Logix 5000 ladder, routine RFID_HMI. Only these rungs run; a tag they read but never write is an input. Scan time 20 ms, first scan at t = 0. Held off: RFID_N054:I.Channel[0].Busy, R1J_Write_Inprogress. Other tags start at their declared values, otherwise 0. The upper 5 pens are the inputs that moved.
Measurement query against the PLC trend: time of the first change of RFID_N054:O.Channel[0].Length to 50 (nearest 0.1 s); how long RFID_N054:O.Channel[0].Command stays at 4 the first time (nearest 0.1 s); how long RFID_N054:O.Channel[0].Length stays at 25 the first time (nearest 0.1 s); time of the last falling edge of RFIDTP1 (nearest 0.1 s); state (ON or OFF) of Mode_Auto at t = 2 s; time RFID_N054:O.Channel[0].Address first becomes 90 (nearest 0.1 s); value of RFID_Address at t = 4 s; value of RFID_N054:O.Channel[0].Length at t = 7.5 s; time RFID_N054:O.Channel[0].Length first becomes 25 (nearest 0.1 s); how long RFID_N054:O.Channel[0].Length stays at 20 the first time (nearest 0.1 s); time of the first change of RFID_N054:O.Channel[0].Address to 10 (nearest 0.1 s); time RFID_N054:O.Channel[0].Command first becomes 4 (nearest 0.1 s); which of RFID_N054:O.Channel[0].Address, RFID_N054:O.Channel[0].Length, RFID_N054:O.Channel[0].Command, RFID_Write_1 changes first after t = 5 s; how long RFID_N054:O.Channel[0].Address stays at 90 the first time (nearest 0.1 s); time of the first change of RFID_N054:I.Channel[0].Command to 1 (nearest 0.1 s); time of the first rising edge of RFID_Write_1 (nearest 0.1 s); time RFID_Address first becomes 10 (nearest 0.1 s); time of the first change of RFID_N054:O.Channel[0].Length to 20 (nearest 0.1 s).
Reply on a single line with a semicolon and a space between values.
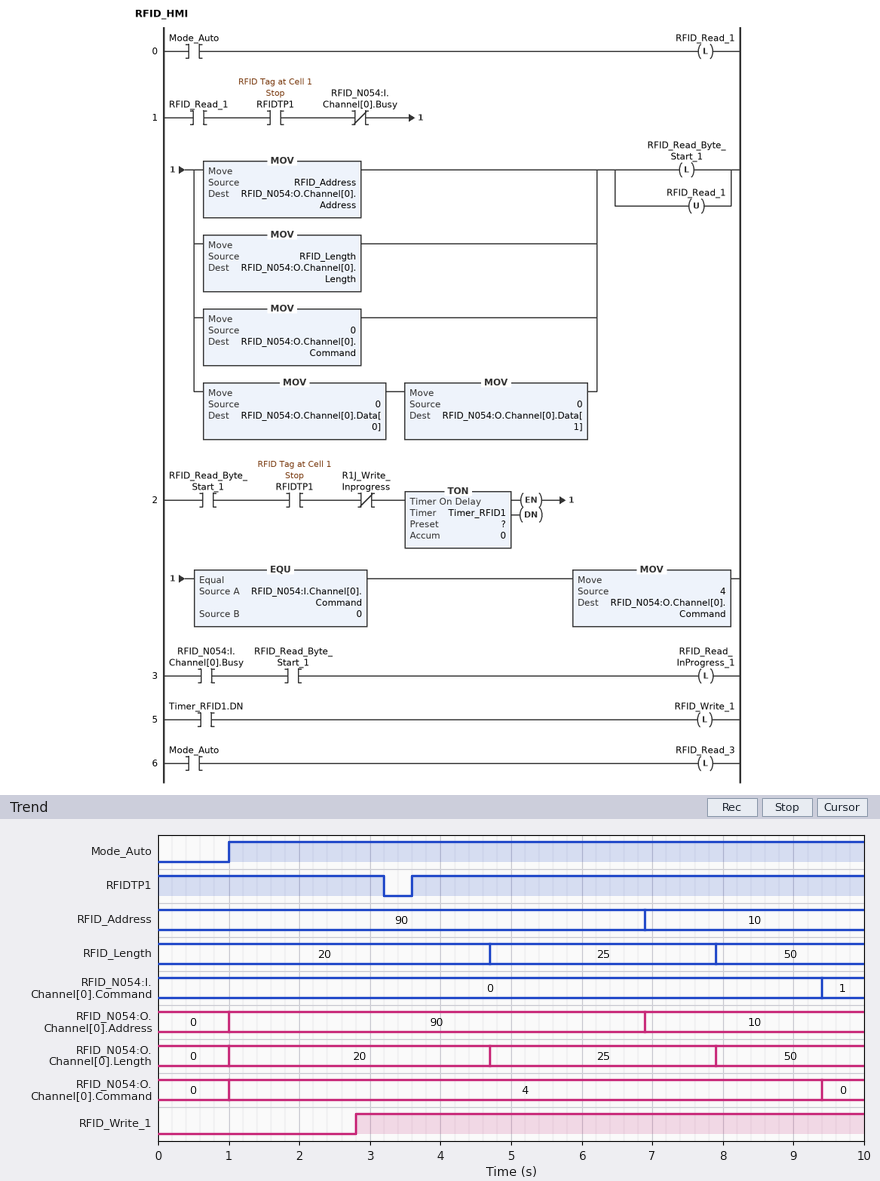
7.9 s; 8.4 s; 3.2 s; 3.2 s; ON; 1.0 s; 90; 25; 4.7 s; 3.7 s; 6.9 s; 1.0 s; RFID_N054:O.Channel[0].Address; 5.9 s; 9.4 s; 2.8 s; 6.9 s; 1.0 s
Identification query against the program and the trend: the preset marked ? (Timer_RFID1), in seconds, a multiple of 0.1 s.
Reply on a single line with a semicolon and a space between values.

1.8 s
